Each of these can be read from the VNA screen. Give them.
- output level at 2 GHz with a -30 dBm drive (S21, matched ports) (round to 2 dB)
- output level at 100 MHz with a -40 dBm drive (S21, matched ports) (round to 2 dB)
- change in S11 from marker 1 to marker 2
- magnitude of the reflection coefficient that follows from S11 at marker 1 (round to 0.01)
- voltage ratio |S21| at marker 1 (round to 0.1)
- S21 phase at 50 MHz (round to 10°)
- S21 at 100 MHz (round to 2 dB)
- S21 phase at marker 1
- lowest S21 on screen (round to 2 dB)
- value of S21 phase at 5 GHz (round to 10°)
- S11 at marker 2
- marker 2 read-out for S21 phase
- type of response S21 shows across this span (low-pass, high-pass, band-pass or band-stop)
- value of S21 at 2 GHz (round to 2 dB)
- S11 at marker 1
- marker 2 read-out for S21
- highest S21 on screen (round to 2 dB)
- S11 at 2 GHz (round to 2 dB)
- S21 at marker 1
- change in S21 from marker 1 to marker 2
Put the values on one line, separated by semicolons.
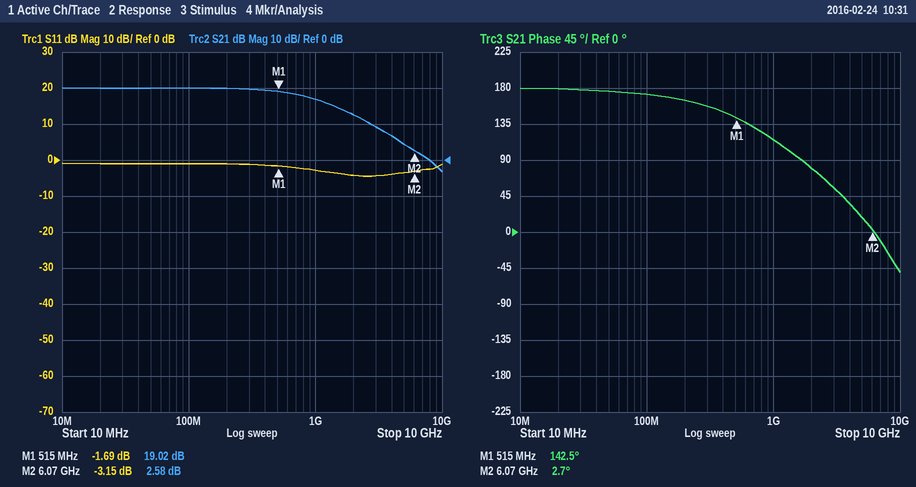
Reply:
-18 dBm; -20 dBm; -1.46 dB; 0.82; 8.9; 180°; 20 dB; 142.5°; -4 dB; 20°; -3.15 dB; 2.7°; low-pass; 12 dB; -1.69 dB; 2.58 dB; 20 dB; -4 dB; 19.02 dB; -16.44 dB
